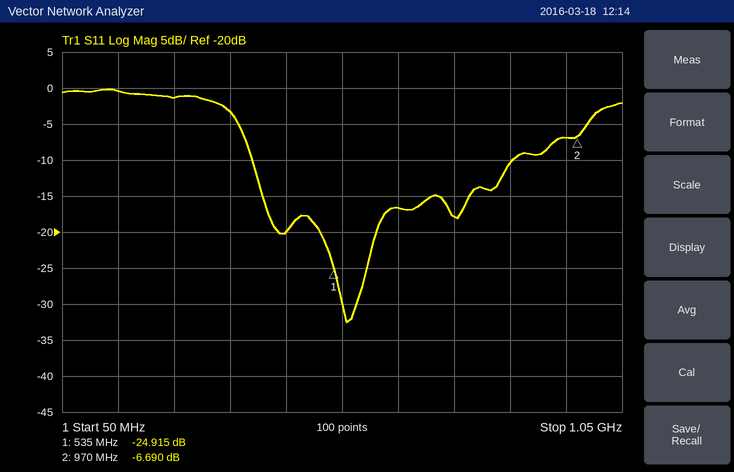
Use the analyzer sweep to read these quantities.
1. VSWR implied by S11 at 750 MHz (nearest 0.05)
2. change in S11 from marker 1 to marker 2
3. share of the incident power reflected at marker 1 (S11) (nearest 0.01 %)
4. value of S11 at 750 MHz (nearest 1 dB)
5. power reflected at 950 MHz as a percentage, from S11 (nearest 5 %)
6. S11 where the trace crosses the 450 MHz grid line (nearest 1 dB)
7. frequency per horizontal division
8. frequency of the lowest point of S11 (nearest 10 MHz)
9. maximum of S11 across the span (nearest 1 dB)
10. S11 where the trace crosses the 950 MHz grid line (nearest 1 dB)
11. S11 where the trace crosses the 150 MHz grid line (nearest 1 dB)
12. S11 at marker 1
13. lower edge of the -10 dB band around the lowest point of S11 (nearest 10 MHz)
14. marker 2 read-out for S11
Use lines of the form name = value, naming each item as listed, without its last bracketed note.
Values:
VSWR implied by S11 at 750 MHz = 1.30
change in S11 from marker 1 to marker 2 = 18.225 dB
share of the incident power reflected at marker 1 (S11) = 0.32 %
value of S11 at 750 MHz = -18 dB
power reflected at 950 MHz as a percentage, from S11 = 20 %
S11 where the trace crosses the 450 MHz grid line = -20 dB
frequency per horizontal division = 100 MHz
frequency of the lowest point of S11 = 560 MHz
maximum of S11 across the span = 0 dB
S11 where the trace crosses the 950 MHz grid line = -7 dB
S11 where the trace crosses the 150 MHz grid line = 0 dB
S11 at marker 1 = -24.915 dB
lower edge of the -10 dB band around the lowest point of S11 = 390 MHz
marker 2 read-out for S11 = -6.690 dB
